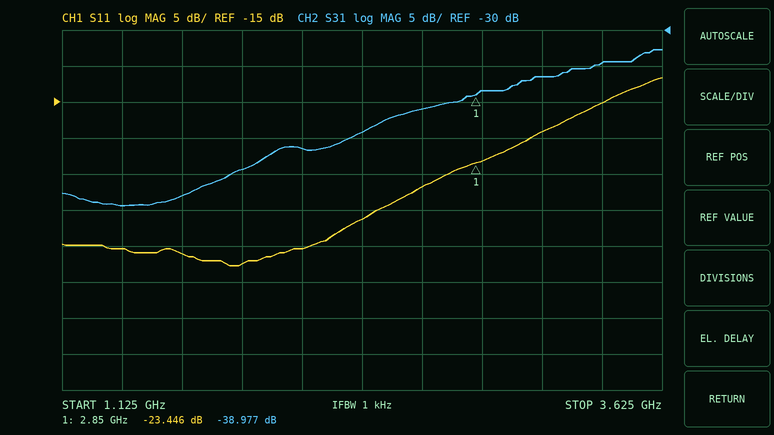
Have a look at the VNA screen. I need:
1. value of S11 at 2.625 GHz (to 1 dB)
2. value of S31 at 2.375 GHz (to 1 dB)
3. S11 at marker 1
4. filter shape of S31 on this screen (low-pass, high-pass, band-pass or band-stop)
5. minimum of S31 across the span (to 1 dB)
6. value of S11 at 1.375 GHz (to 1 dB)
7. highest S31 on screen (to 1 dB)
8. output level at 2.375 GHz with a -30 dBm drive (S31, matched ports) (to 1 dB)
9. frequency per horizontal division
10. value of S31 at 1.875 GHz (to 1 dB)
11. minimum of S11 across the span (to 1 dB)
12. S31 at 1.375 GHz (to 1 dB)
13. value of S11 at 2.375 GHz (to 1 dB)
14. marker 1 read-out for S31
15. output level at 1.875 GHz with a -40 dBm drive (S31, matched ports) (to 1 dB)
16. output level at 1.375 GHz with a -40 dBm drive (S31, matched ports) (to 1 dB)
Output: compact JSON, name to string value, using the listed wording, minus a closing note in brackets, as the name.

{"value of S11 at 2.625 GHz": "-27 dB", "value of S31 at 2.375 GHz": "-44 dB", "S11 at marker 1": "-23.446 dB", "filter shape of S31 on this screen": "high-pass", "minimum of S31 across the span": "-54 dB", "value of S11 at 1.375 GHz": "-35 dB", "highest S31 on screen": "-33 dB", "output level at 2.375 GHz with a -30 dBm drive (S31, matched ports)": "-74 dBm", "frequency per horizontal division": "250 MHz", "value of S31 at 1.875 GHz": "-49 dB", "minimum of S11 across the span": "-38 dB", "S31 at 1.375 GHz": "-54 dB", "value of S11 at 2.375 GHz": "-31 dB", "marker 1 read-out for S31": "-38.977 dB", "output level at 1.875 GHz with a -40 dBm drive (S31, matched ports)": "-89 dBm", "output level at 1.375 GHz with a -40 dBm drive (S31, matched ports)": "-94 dBm"}
